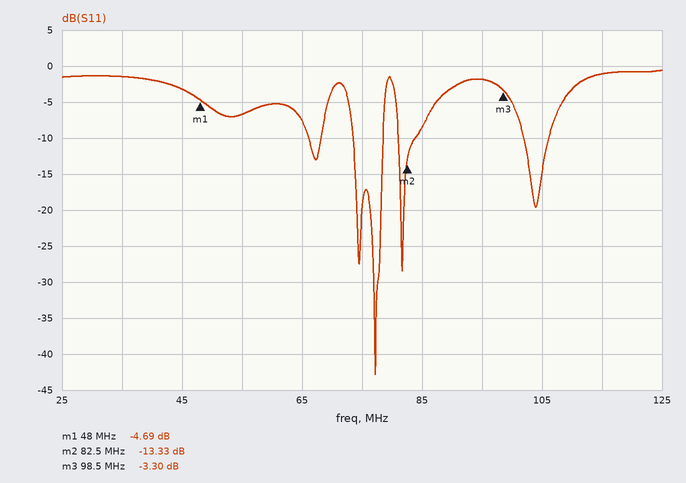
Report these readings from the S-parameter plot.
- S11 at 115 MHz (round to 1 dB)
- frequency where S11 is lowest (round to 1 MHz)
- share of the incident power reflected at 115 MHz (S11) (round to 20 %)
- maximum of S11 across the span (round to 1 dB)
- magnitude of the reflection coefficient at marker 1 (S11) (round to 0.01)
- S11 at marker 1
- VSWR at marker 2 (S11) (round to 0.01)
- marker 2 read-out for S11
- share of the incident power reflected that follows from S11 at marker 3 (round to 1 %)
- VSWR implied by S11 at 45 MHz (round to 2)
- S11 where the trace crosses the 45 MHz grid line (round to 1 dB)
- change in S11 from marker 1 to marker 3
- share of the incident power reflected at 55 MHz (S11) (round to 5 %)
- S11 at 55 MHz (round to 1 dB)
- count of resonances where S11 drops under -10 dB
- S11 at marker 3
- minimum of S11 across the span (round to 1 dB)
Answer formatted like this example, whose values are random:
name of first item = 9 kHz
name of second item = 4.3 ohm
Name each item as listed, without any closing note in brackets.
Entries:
S11 at 115 MHz = -1 dB
frequency where S11 is lowest = 77 MHz
share of the incident power reflected at 115 MHz (S11) = 80 %
maximum of S11 across the span = -1 dB
magnitude of the reflection coefficient at marker 1 (S11) = 0.58
S11 at marker 1 = -4.69 dB
VSWR at marker 2 (S11) = 1.55
marker 2 read-out for S11 = -13.33 dB
share of the incident power reflected that follows from S11 at marker 3 = 47 %
VSWR implied by S11 at 45 MHz = 6
S11 where the trace crosses the 45 MHz grid line = -3 dB
change in S11 from marker 1 to marker 3 = 1.39 dB
share of the incident power reflected at 55 MHz (S11) = 20 %
S11 at 55 MHz = -7 dB
count of resonances where S11 drops under -10 dB = 5
S11 at marker 3 = -3.30 dB
minimum of S11 across the span = -43 dB
